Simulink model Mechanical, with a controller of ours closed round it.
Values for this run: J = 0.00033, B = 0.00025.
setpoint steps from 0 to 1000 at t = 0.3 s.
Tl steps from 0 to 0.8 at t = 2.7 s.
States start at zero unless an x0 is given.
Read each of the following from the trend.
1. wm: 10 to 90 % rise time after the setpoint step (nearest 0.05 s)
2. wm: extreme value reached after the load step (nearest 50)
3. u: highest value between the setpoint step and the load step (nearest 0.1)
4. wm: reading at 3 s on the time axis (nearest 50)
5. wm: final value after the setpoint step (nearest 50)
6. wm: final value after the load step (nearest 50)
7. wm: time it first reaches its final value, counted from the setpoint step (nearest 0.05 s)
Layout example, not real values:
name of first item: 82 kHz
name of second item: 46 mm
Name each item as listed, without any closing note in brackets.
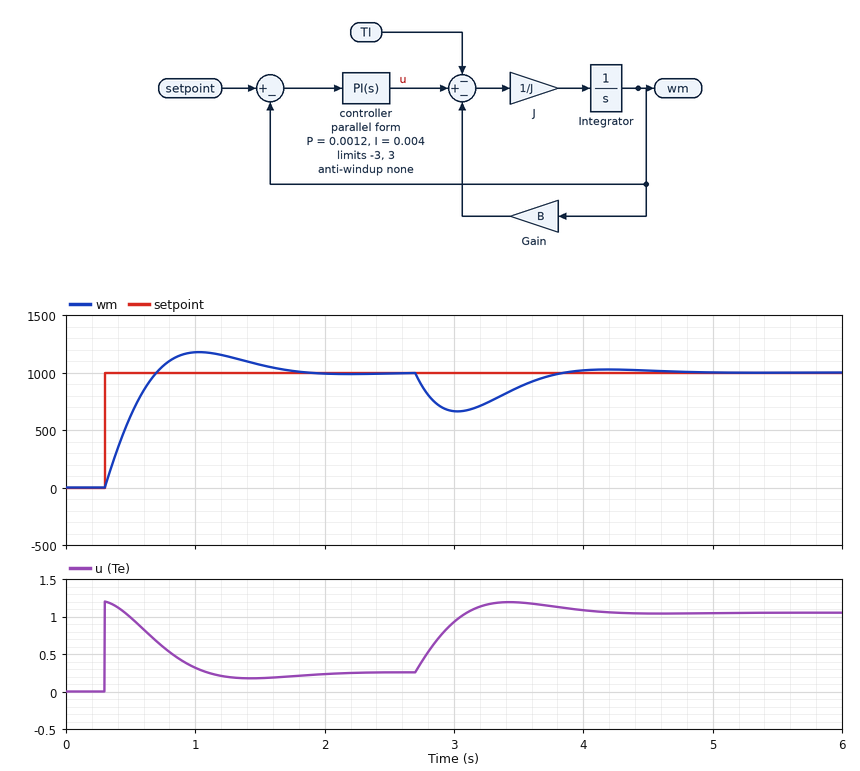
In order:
wm: 10 to 90 % rise time after the setpoint step: 0.30 s
wm: extreme value reached after the load step: 650
u: highest value between the setpoint step and the load step: 1.2
wm: reading at 3 s on the time axis: 650
wm: final value after the setpoint step: 1000
wm: final value after the load step: 1000
wm: time it first reaches its final value, counted from the setpoint step: 0.40 s
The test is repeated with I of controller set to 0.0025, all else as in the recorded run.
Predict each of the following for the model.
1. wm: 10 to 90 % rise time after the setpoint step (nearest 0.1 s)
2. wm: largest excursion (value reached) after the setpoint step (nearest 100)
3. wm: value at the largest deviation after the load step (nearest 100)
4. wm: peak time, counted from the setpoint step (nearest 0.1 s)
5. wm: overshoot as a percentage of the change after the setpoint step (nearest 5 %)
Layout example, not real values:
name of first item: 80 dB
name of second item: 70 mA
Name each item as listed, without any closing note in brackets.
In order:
wm: 10 to 90 % rise time after the setpoint step: 0.4 s
wm: largest excursion (value reached) after the setpoint step: 1100
wm: value at the largest deviation after the load step: 600
wm: peak time, counted from the setpoint step: 0.9 s
wm: overshoot as a percentage of the change after the setpoint step: 10 %
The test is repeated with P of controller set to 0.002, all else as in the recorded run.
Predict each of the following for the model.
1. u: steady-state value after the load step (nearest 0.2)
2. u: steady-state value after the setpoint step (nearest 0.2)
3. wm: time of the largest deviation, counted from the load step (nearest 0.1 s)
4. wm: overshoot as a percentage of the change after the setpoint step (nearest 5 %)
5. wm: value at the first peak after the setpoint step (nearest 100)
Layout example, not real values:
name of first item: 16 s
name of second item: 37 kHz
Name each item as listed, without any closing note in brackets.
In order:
u: steady-state value after the load step: 1.0
u: steady-state value after the setpoint step: 0.2
wm: time of the largest deviation, counted from the load step: 0.3 s
wm: overshoot as a percentage of the change after the setpoint step: 10 %
wm: value at the first peak after the setpoint step: 1100
